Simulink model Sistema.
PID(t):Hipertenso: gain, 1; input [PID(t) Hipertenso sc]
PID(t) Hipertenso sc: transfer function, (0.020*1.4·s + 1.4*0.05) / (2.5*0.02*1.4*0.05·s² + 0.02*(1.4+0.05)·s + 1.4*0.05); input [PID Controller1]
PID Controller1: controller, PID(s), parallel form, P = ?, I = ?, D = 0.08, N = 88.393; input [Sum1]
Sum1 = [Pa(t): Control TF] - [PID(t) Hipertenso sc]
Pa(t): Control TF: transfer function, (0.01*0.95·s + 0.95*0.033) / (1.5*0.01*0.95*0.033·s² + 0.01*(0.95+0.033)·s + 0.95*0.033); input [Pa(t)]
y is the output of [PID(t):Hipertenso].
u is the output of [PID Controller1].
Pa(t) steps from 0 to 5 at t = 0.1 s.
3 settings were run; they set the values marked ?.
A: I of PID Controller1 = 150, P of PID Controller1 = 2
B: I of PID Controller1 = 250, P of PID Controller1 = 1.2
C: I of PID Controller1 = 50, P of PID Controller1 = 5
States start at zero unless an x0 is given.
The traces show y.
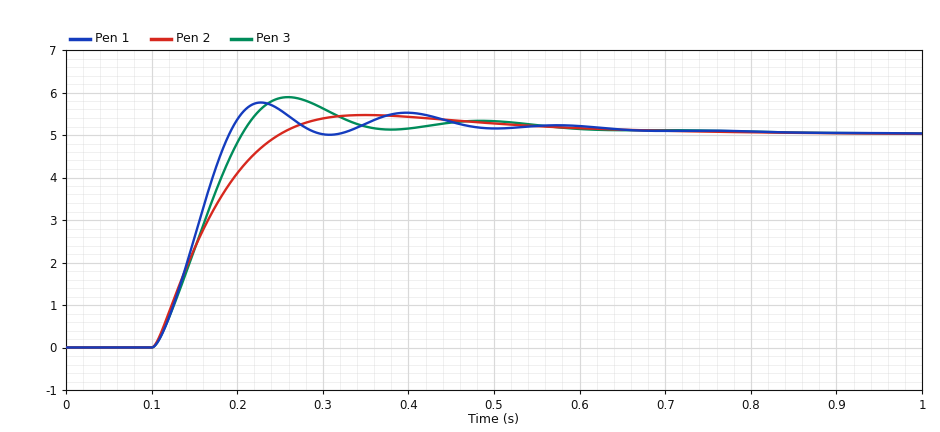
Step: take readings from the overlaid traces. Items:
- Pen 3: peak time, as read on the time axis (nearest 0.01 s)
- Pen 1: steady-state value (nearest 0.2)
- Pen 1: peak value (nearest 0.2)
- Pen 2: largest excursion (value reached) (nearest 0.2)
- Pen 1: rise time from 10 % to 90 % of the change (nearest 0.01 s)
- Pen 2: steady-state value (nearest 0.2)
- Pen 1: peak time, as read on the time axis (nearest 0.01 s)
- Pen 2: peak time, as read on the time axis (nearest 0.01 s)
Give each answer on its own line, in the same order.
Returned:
0.26 s
5.0
5.8
5.4
0.06 s
5.0
0.23 s
0.35 s
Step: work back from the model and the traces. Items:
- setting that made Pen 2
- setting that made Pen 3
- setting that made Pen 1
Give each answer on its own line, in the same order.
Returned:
C
A
B
